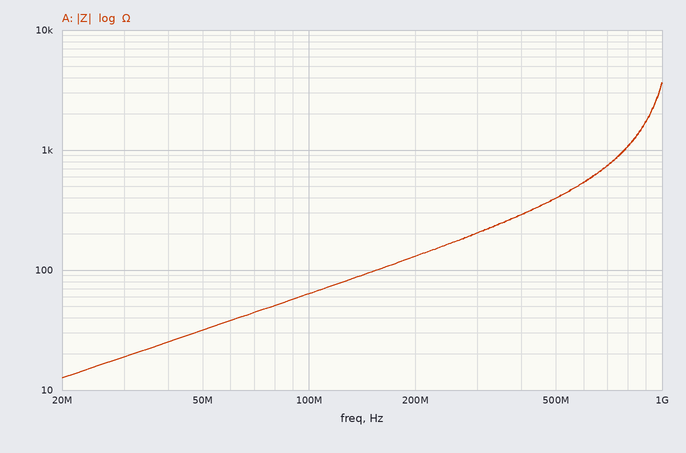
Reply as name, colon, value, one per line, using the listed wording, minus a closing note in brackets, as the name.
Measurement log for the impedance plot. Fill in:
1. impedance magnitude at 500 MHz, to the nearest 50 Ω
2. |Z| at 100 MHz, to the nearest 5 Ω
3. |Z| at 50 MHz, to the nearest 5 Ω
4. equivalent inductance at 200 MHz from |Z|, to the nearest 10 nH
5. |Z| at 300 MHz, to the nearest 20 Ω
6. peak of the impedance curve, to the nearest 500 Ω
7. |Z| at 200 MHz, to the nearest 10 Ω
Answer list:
impedance magnitude at 500 MHz, to the nearest 50 Ω: 400 Ω
|Z| at 100 MHz, to the nearest 5 Ω: 65 Ω
|Z| at 50 MHz, to the nearest 5 Ω: 30 Ω
equivalent inductance at 200 MHz from |Z|, to the nearest 10 nH: 100 nH
|Z| at 300 MHz, to the nearest 20 Ω: 200 Ω
peak of the impedance curve, to the nearest 500 Ω: 3.5 kΩ
|Z| at 200 MHz, to the nearest 10 Ω: 130 Ω
